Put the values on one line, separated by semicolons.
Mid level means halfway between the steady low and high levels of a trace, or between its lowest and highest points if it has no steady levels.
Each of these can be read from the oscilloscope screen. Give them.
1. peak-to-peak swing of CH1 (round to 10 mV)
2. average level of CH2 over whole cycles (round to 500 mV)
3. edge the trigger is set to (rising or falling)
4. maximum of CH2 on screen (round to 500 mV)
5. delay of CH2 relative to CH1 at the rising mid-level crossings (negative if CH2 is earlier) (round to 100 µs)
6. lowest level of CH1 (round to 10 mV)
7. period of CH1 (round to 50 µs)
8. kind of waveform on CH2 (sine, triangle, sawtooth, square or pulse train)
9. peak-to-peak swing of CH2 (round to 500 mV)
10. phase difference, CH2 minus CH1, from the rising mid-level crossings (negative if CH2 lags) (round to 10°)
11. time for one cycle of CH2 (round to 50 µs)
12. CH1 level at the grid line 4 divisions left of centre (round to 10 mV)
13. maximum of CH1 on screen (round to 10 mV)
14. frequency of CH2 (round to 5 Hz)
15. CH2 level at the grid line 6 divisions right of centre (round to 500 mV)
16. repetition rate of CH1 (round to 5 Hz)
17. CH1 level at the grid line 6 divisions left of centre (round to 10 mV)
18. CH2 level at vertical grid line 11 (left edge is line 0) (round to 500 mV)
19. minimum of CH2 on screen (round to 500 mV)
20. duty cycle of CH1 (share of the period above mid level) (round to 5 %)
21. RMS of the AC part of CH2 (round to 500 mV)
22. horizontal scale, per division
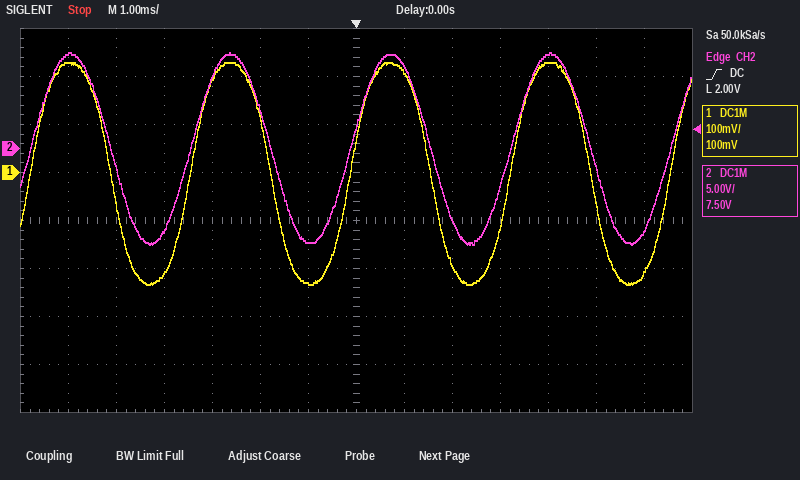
460 mV; 0.0 V; rising; 10.0 V; 0.0 ms; -230 mV; 3.35 ms; sine; 20.0 V; 0°; 3.35 ms; -210 mV; 230 mV; 300 Hz; -8.5 V; 300 Hz; 230 mV; 10.0 V; -10.0 V; 50 %; 7.0 V; 1 ms
